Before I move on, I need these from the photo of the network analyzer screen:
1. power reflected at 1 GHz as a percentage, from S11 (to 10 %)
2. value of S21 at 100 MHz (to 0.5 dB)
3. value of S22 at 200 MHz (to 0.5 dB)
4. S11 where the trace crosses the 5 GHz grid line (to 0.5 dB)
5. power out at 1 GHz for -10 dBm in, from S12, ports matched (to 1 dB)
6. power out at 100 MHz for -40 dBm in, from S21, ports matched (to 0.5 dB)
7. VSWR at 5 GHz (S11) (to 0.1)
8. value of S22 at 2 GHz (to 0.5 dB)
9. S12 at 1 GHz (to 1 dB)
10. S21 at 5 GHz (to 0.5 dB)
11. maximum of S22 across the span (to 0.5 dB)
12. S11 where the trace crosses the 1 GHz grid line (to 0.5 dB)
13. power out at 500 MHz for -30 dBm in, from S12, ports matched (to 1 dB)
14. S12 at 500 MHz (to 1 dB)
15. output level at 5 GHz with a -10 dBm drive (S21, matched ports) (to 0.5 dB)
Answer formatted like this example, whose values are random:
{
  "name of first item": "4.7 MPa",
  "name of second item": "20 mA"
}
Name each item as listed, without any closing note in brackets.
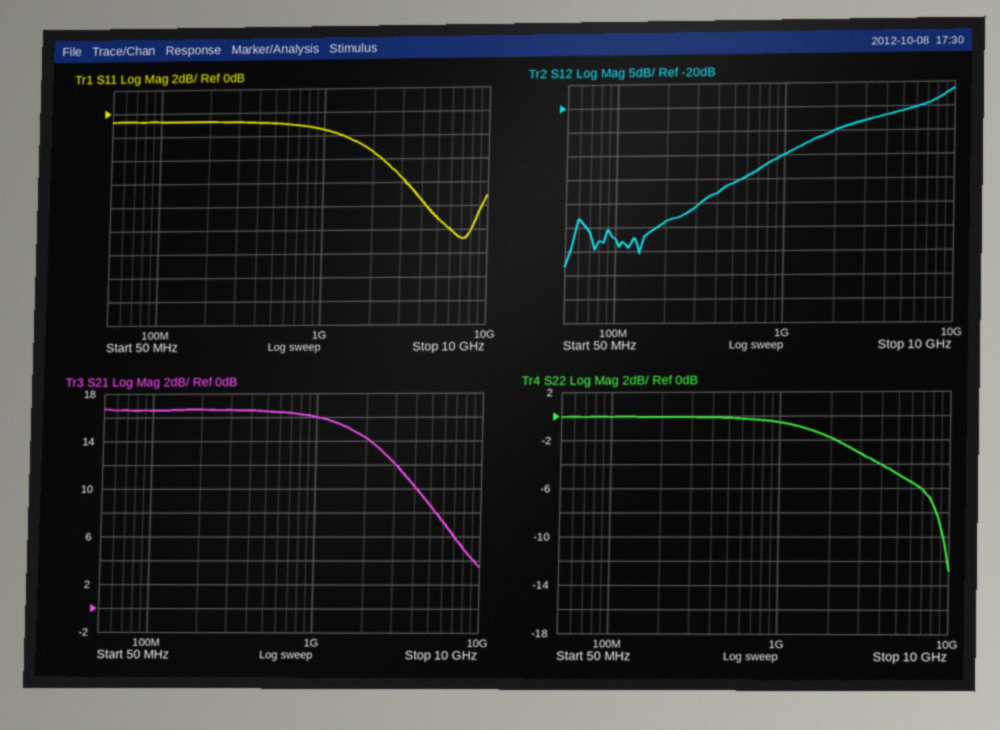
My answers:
{
  "power reflected at 1 GHz as a percentage, from S11": "70 %",
  "value of S21 at 100 MHz": "16.5 dB",
  "value of S22 at 200 MHz": "0.0 dB",
  "S11 where the trace crosses the 5 GHz grid line": "-9.0 dB",
  "power out at 1 GHz for -10 dBm in, from S12, ports matched": "-40 dBm",
  "power out at 100 MHz for -40 dBm in, from S21, ports matched": "-23.5 dBm",
  "VSWR at 5 GHz (S11)": "2.1",
  "value of S22 at 2 GHz": "-2.0 dB",
  "S12 at 1 GHz": "-30 dB",
  "S21 at 5 GHz": "8.5 dB",
  "maximum of S22 across the span": "0.0 dB",
  "S11 where the trace crosses the 1 GHz grid line": "-1.5 dB",
  "power out at 500 MHz for -30 dBm in, from S12, ports matched": "-66 dBm",
  "S12 at 500 MHz": "-36 dB",
  "output level at 5 GHz with a -10 dBm drive (S21, matched ports)": "-1.5 dBm"
}
